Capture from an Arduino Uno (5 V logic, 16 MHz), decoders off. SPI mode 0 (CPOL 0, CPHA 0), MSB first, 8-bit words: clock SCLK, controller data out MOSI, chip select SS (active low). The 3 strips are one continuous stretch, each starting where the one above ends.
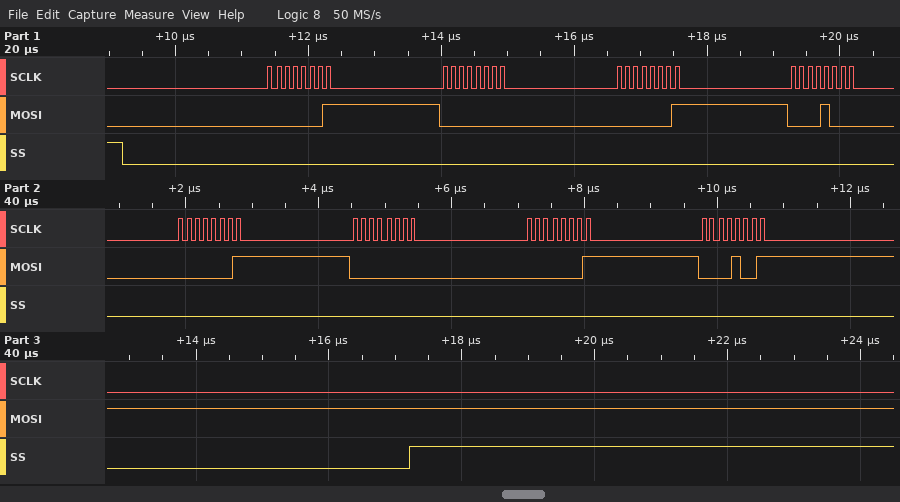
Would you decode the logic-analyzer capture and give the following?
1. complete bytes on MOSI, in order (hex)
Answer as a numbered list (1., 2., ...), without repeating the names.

1. 01 00 01 08 01 00 01 09
